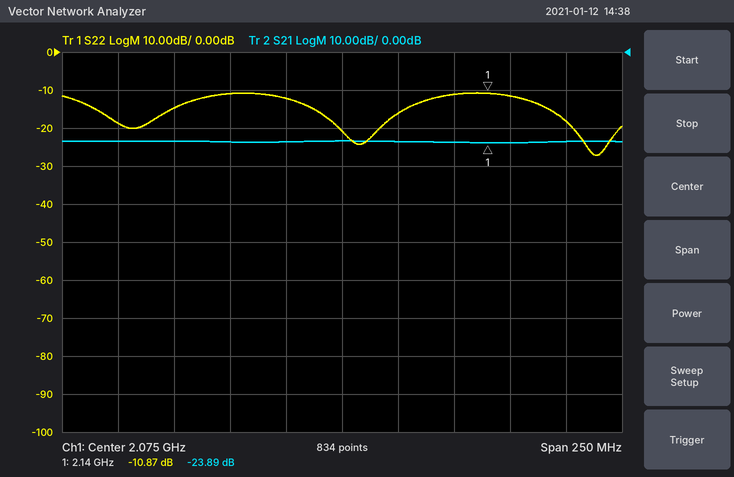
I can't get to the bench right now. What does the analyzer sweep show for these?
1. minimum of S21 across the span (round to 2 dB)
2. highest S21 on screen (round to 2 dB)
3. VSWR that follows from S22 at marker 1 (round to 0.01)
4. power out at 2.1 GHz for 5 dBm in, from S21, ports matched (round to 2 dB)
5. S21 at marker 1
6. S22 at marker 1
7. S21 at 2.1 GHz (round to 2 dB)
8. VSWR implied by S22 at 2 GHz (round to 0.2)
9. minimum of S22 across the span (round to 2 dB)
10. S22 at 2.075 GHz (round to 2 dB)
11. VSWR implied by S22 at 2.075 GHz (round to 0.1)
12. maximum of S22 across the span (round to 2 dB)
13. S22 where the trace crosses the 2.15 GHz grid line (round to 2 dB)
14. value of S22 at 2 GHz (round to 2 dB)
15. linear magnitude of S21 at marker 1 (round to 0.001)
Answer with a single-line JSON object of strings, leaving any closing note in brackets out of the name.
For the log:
{"minimum of S21 across the span": "-24 dB", "highest S21 on screen": "-24 dB", "VSWR that follows from S22 at marker 1": "1.80", "power out at 2.1 GHz for 5 dBm in, from S21, ports matched": "-18 dBm", "S21 at marker 1": "-23.89 dB", "S22 at marker 1": "-10.87 dB", "S21 at 2.1 GHz": "-24 dB", "VSWR implied by S22 at 2 GHz": "1.4", "minimum of S22 across the span": "-28 dB", "S22 at 2.075 GHz": "-20 dB", "VSWR implied by S22 at 2.075 GHz": "1.2", "maximum of S22 across the span": "-10 dB", "S22 where the trace crosses the 2.15 GHz grid line": "-12 dB", "value of S22 at 2 GHz": "-14 dB", "linear magnitude of S21 at marker 1": "0.064"}
